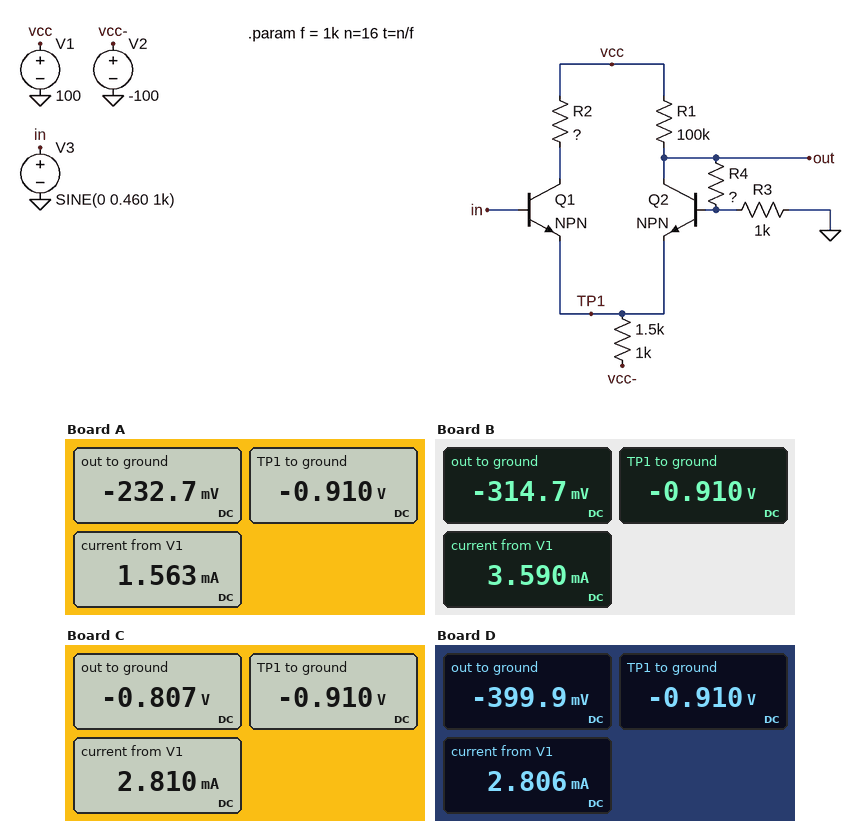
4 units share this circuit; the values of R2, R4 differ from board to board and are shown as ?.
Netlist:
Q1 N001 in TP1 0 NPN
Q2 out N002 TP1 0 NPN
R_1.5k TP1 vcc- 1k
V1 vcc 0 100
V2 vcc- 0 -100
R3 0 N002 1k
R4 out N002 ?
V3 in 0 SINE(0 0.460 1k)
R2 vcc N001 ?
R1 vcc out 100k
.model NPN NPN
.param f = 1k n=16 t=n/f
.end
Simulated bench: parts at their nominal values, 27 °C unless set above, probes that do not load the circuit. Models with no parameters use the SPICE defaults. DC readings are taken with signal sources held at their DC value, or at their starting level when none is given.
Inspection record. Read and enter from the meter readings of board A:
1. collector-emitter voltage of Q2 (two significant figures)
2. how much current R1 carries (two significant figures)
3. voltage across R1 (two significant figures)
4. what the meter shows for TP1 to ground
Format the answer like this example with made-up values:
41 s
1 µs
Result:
680 mV
1.0 mA
100 V
-0.910 V
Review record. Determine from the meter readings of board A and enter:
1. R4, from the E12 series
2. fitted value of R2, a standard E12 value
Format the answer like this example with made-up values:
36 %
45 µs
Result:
820 Ω
180 kΩ
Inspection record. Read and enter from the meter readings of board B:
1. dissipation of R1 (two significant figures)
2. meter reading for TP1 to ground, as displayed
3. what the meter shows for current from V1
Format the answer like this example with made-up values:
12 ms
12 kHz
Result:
100 mW
-0.910 V
3.590 mA
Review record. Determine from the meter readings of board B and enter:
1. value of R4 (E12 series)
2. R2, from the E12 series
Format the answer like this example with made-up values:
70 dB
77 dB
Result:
1.5 kΩ
39 kΩ
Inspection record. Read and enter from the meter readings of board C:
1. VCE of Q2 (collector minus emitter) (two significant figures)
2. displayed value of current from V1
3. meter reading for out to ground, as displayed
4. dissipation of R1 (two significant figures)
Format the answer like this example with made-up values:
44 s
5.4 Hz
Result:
100 mV
2.810 mA
-0.807 V
100 mW
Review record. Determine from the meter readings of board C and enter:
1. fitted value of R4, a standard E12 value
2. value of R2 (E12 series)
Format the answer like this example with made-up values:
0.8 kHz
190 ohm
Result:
6.8 kΩ
56 kΩ
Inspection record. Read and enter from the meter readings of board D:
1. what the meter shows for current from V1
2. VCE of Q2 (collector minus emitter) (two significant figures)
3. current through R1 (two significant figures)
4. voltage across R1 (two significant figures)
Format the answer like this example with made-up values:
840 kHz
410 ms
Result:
2.806 mA
510 mV
1.0 mA
100 V
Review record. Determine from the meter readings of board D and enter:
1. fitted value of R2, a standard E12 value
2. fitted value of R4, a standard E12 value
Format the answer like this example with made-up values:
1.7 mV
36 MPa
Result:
56 kΩ
2.2 kΩ
